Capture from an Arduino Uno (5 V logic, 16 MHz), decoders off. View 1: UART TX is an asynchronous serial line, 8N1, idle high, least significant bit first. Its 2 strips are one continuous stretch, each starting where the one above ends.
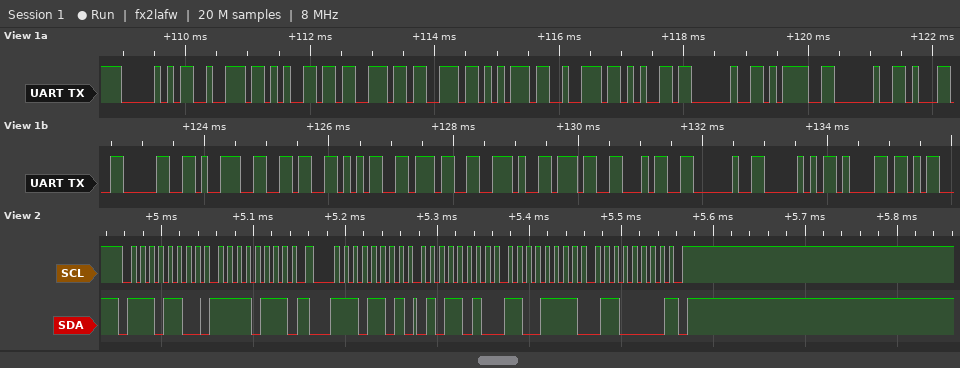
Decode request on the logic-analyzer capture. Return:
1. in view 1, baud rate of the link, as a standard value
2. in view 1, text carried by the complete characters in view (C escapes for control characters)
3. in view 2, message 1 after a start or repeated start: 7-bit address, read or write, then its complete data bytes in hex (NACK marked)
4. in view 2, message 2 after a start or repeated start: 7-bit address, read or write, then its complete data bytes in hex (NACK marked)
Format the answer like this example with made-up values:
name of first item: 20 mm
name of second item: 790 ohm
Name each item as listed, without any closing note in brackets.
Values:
in view 1, baud rate of the link, as a standard value: 9600 baud
in view 1, text carried by the complete characters in view: "Pressure = 109657.74 Pa"
in view 2, message 1 after a start or repeated start: 7-bit address, read or write, then its complete data bytes in hex: 0x76 write: F7
in view 2, message 2 after a start or repeated start: 7-bit address, read or write, then its complete data bytes in hex: 0x76 read: 5A CF 60 NACK
